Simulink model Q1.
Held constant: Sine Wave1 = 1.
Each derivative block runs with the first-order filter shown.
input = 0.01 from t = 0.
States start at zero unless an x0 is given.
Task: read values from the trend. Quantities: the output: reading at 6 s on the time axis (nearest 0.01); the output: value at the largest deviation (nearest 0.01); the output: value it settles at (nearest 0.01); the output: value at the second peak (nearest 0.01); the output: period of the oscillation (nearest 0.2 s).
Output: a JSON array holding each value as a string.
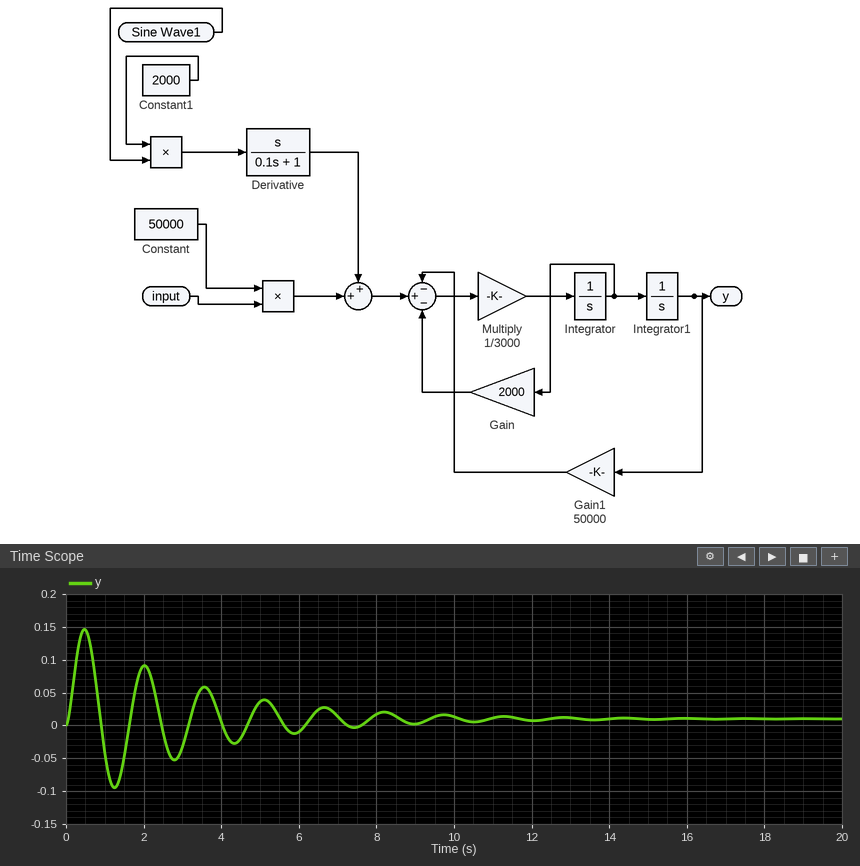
["-0.01", "0.15", "0.01", "0.09", "1.6 s"]
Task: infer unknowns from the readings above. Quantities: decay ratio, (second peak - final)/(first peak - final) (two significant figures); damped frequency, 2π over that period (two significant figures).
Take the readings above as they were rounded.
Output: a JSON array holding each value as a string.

["0.57", "3.9 rad/s"]
